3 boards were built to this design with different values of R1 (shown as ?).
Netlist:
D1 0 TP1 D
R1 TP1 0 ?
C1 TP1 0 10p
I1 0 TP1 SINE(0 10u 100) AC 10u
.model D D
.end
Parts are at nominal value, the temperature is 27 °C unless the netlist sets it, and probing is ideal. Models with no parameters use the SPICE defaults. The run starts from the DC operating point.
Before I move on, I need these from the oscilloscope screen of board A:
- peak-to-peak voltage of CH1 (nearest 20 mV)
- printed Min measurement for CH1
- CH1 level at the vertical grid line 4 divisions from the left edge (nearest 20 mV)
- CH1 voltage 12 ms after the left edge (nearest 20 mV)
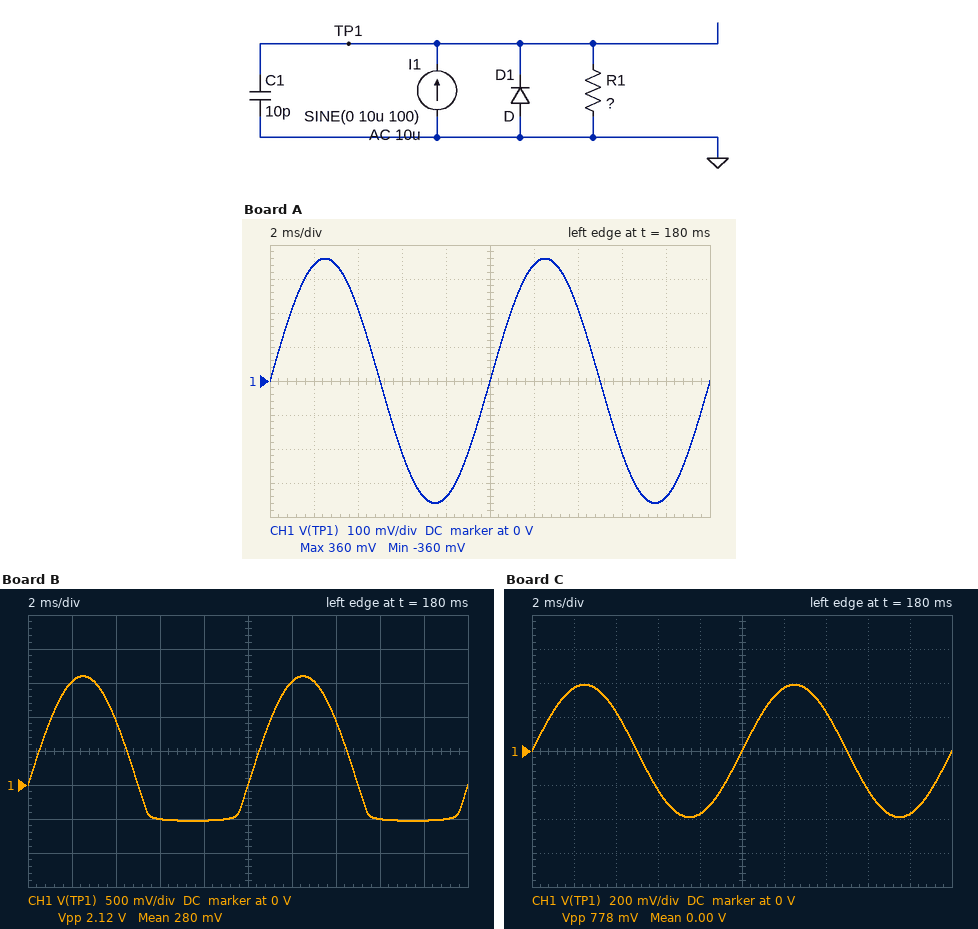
720 mV
-360 mV
-340 mV
340 mV
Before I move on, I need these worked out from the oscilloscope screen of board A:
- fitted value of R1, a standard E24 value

36 kΩ
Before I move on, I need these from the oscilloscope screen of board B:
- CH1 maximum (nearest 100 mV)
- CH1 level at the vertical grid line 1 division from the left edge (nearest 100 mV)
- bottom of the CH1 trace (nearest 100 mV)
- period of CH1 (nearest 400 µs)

1.6 V
1.5 V
-500 mV
10.0 ms
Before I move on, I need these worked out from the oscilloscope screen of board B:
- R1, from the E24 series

160 kΩ
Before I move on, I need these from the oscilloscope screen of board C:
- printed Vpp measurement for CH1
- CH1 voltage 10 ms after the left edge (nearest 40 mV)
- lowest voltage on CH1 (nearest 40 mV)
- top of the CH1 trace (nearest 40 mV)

778 mV
0 V
-400 mV
400 mV
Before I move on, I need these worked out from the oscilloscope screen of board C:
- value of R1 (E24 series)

39 kΩ
